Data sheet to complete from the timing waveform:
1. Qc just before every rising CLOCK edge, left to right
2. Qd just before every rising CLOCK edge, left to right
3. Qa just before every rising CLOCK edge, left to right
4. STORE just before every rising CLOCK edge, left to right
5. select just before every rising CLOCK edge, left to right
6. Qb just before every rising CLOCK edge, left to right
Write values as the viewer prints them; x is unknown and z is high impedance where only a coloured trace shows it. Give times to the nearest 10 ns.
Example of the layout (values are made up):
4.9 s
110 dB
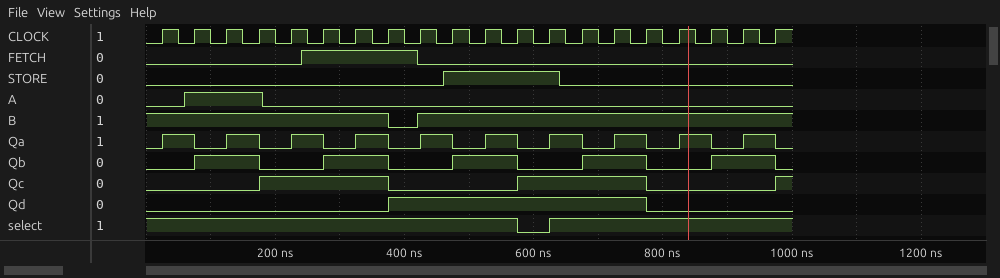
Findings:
0 0 0 0 1 1 1 1 0 0 0 0 1 1 1 1 0 0 0 0
0 0 0 0 0 0 0 0 1 1 1 1 1 1 1 1 0 0 0 0
0 1 0 1 0 1 0 1 0 1 0 1 0 1 0 1 0 1 0 1
0 0 0 0 0 0 0 0 0 1 1 1 1 0 0 0 0 0 0 0
1 1 1 1 1 1 1 1 1 1 1 1 0 1 1 1 1 1 1 1
0 0 1 1 0 0 1 1 0 0 1 1 0 0 1 1 0 0 1 1
